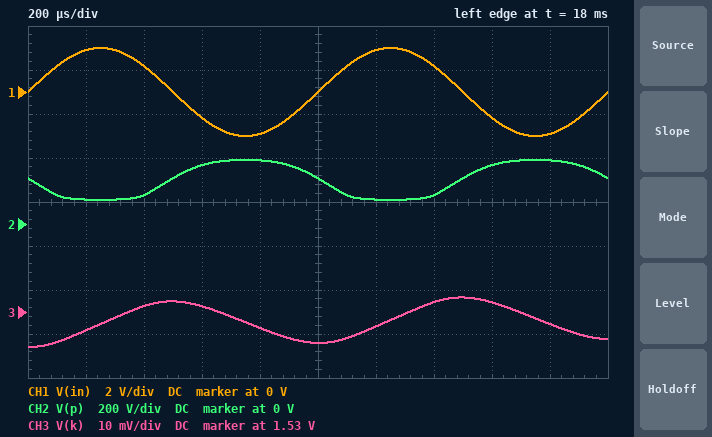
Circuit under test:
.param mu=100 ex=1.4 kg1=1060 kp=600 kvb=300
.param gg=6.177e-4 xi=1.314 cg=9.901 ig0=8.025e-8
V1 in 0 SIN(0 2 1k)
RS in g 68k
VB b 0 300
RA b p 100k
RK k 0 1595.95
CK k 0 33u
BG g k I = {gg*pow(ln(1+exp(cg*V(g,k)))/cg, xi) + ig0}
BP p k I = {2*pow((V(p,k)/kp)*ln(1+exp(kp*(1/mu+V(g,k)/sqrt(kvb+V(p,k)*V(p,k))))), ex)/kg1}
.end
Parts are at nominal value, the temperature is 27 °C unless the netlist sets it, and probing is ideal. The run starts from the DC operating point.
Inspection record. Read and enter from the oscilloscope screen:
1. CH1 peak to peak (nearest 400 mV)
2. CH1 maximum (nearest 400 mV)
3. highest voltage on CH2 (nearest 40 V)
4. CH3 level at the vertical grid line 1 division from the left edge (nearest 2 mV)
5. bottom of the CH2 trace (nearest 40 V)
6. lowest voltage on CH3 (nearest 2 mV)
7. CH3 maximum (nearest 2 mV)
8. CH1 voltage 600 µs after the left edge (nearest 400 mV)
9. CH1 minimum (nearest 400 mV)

4.0 V
2.0 V
280 V
1.526 V
120 V
1.522 V
1.534 V
-1.2 V
-2.0 V
